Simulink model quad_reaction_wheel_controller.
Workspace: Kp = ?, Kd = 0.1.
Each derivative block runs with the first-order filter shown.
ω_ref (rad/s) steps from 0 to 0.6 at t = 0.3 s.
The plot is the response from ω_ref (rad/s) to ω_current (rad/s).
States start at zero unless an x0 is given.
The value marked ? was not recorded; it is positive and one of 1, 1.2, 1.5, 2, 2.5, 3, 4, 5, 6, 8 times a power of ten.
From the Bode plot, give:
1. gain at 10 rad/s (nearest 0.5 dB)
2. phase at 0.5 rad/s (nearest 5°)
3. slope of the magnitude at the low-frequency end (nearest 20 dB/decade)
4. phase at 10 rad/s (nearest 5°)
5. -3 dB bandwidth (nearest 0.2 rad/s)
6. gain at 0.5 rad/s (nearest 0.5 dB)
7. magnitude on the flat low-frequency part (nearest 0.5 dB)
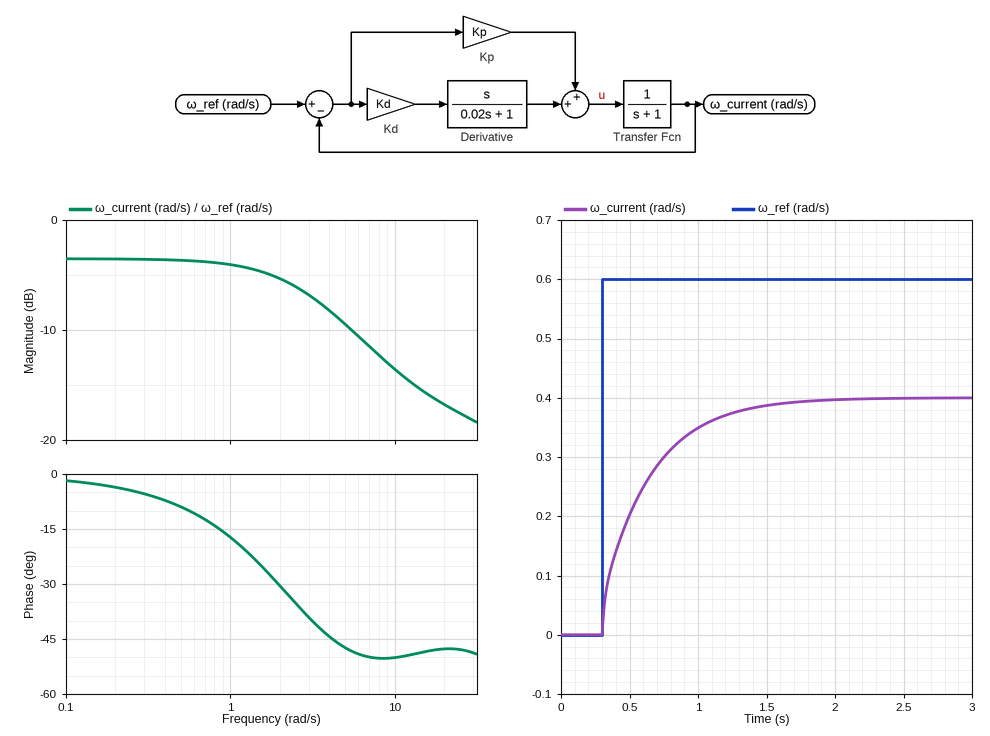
-13.5 dB
-10°
0 dB/decade
-50°
2.8 rad/s
-3.5 dB
-3.5 dB
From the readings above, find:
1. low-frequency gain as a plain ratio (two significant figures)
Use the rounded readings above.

0.67
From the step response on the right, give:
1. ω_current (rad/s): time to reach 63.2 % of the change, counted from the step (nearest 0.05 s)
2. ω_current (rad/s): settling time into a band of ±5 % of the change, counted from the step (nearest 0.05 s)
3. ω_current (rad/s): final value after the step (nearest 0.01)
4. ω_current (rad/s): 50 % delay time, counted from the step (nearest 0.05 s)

0.30 s
1.05 s
0.40
0.20 s
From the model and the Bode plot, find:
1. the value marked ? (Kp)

2
